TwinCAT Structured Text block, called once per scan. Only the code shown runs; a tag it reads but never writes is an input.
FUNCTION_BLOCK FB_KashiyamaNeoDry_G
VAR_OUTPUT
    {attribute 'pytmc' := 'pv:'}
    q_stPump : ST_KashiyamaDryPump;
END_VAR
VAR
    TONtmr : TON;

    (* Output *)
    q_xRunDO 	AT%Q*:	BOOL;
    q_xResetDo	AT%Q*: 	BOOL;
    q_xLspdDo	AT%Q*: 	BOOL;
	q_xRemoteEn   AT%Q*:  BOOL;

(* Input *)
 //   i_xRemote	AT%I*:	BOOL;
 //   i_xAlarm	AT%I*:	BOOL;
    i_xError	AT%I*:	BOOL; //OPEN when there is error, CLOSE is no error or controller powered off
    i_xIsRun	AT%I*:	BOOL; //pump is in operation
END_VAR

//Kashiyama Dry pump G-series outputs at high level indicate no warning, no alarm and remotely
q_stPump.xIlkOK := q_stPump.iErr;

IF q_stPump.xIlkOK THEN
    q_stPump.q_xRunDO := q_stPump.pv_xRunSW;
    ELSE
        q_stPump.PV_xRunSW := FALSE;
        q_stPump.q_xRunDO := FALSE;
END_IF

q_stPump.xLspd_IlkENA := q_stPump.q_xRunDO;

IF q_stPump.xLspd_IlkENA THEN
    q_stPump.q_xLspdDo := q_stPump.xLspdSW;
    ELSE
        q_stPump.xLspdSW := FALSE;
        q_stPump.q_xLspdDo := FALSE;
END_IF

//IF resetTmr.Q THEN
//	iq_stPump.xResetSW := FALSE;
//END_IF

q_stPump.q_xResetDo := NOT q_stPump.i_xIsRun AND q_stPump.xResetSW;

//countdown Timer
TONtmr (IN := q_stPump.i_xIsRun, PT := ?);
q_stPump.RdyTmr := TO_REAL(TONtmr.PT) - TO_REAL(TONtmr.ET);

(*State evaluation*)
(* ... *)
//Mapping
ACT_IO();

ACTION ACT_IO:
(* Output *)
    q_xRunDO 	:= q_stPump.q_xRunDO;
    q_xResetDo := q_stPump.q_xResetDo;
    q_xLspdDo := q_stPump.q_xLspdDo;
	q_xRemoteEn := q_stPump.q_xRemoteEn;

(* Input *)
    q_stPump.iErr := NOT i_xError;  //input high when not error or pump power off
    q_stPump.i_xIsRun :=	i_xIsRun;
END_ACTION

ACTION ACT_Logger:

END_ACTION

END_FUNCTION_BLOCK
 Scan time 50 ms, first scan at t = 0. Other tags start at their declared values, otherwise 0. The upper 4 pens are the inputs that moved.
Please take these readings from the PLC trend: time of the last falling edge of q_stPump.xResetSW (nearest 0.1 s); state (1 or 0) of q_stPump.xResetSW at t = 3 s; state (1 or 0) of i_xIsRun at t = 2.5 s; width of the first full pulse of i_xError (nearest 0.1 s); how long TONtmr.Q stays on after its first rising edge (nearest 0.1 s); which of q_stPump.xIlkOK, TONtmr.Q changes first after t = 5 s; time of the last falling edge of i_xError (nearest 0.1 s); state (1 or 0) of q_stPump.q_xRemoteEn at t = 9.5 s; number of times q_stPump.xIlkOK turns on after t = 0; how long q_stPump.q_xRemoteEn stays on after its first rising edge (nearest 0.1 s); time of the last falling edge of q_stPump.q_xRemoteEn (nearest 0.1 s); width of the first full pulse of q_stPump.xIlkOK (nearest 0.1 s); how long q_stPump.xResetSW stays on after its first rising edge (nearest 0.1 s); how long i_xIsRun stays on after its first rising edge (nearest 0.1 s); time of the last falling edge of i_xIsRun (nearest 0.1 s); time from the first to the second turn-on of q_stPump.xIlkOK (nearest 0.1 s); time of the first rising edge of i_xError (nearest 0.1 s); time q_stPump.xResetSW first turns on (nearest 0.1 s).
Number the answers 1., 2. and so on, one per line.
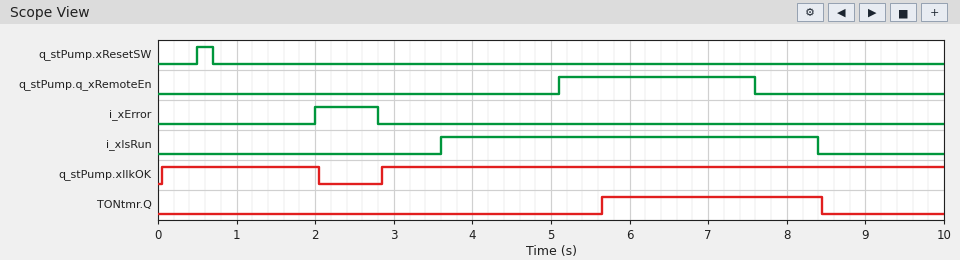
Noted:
1. 0.7 s
2. 0
3. 0
4. 0.8 s
5. 2.8 s
6. TONtmr.Q
7. 2.8 s
8. 0
9. 2
10. 2.5 s
11. 7.6 s
12. 2.0 s
13. 0.2 s
14. 4.8 s
15. 8.4 s
16. 2.8 s
17. 2.0 s
18. 0.5 s
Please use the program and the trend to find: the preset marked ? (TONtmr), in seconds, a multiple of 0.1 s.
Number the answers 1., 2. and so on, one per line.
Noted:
1. 2.0 s
